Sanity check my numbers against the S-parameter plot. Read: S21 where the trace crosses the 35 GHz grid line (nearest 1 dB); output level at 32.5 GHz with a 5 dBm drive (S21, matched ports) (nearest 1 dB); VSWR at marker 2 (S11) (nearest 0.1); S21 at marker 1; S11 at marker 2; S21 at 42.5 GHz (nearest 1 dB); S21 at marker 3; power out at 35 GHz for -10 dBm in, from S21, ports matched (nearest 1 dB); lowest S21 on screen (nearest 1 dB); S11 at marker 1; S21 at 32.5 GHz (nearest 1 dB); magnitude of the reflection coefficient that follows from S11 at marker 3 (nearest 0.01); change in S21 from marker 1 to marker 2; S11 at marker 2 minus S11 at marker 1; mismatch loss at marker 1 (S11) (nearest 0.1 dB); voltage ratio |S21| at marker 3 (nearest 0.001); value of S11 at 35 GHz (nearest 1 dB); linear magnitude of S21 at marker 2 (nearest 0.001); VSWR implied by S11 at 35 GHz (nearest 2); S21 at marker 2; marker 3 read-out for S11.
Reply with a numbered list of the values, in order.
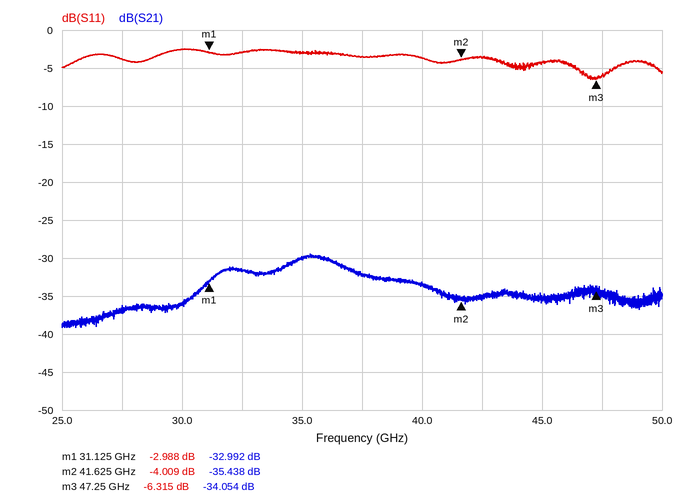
1. -30 dB
2. -27 dBm
3. 4.4
4. -32.992 dB
5. -4.009 dB
6. -35 dB
7. -34.054 dB
8. -40 dBm
9. -39 dB
10. -2.988 dB
11. -32 dB
12. 0.48
13. -2.446 dB
14. -1.021 dB
15. 3.0 dB
16. 0.020
17. -3 dB
18. 0.017
19. 6
20. -35.438 dB
21. -6.315 dB
